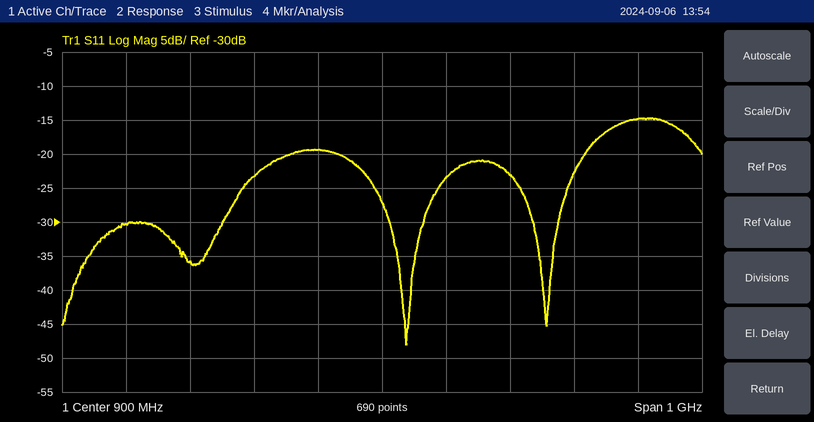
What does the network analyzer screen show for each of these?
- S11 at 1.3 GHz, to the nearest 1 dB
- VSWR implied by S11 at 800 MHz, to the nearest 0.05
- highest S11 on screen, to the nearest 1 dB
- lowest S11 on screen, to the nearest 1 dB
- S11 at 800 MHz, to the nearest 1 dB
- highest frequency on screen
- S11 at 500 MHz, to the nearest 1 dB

-15 dB
1.25
-15 dB
-48 dB
-19 dB
1.4 GHz
-30 dB
